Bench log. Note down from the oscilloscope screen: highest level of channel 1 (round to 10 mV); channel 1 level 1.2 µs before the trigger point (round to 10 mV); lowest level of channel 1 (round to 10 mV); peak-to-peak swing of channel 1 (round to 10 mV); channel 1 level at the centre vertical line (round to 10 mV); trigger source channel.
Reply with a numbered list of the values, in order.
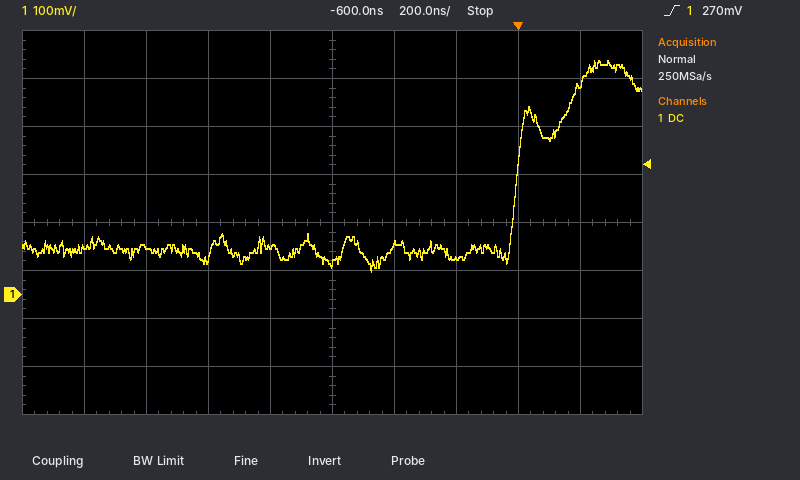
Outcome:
1. 490 mV
2. 100 mV
3. 50 mV
4. 440 mV
5. 60 mV
6. channel 1
